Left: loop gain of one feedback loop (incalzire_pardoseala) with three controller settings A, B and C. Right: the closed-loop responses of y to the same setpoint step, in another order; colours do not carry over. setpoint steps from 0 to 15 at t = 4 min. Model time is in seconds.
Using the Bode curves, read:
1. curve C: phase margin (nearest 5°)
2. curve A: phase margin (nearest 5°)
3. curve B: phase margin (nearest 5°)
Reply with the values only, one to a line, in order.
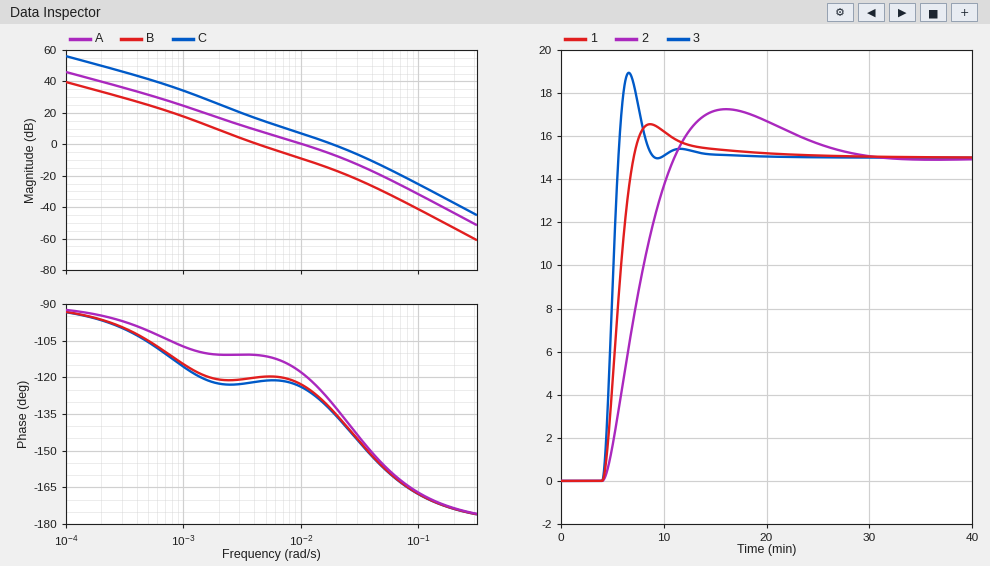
45°
60°
60°
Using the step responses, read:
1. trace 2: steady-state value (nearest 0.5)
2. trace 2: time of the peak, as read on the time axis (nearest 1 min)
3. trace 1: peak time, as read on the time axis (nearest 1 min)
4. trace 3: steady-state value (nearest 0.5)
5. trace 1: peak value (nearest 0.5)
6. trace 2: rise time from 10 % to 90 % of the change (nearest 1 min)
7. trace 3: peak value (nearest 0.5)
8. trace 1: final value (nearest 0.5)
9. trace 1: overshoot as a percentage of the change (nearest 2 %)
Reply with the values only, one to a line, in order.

15.0
16 min
9 min
15.0
16.5
5 min
19.0
15.0
10 %
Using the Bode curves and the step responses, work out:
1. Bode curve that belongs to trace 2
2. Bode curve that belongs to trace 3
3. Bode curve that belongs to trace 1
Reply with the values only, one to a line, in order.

B
C
A
